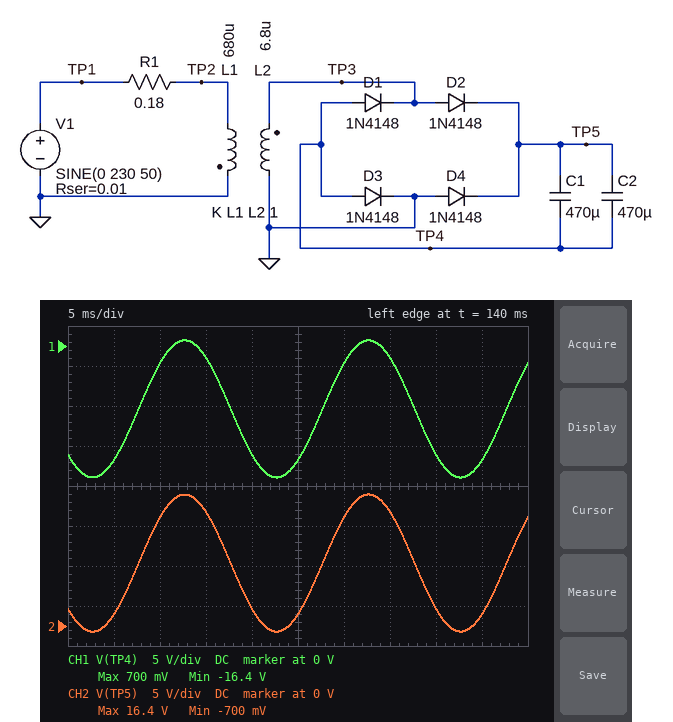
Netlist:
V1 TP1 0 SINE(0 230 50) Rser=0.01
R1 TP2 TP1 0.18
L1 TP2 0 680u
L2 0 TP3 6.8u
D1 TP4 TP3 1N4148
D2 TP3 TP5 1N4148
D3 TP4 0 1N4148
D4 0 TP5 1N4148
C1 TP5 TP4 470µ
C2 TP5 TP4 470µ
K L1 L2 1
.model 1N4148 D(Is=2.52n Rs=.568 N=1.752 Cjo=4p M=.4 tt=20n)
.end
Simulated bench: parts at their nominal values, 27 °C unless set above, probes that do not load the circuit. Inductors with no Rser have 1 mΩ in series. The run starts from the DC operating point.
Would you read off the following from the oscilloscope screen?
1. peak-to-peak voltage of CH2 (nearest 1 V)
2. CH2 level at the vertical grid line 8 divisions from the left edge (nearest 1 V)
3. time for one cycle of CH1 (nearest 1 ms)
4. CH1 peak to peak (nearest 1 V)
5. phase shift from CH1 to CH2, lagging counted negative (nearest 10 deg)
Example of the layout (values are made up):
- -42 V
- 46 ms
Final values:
- 17 V
- 2 V
- 20 ms
- 17 V
- 0 deg
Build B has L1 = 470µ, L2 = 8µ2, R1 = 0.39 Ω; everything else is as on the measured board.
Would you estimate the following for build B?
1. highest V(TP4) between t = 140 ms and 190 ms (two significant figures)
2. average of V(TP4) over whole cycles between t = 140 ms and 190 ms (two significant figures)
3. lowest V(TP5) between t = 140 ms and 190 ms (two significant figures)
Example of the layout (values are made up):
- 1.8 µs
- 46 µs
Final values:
- 700 mV
- -4.6 V
- -700 mV
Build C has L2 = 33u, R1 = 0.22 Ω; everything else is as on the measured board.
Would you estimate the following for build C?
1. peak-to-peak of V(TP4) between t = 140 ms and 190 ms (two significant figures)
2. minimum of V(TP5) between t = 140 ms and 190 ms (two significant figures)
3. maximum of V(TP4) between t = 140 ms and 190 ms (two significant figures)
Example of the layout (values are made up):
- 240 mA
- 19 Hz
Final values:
- 34 V
- -750 mV
- 740 mV
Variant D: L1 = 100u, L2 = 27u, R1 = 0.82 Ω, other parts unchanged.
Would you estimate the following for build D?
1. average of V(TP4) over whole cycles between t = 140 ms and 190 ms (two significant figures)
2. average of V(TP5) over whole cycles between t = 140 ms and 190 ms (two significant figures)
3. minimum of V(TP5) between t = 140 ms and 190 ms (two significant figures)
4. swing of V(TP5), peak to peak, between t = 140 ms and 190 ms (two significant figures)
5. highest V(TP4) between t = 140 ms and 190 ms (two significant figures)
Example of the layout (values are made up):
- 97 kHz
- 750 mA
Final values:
- -1.6 V
- 1.6 V
- -670 mV
- 4.5 V
- 670 mV
